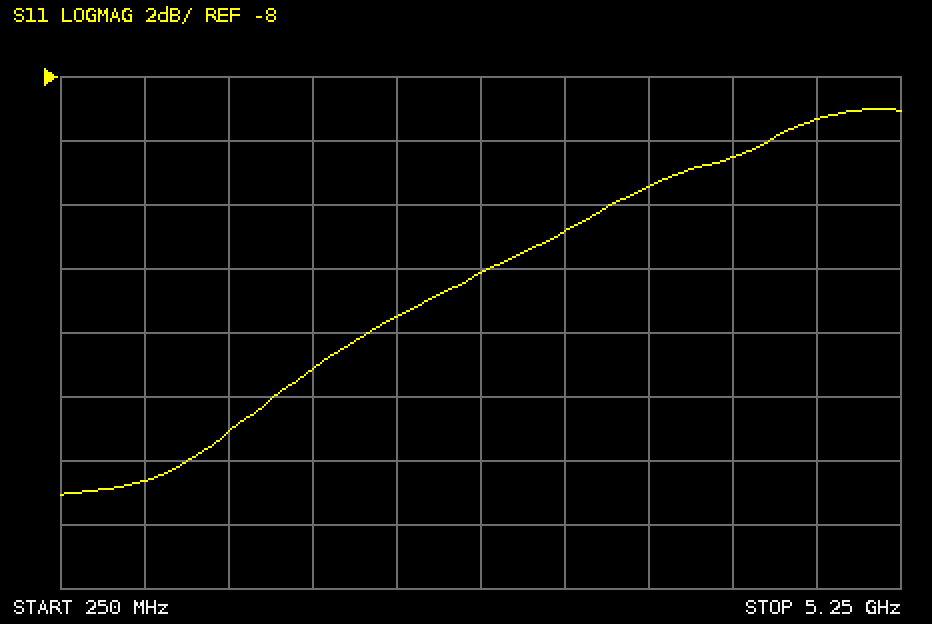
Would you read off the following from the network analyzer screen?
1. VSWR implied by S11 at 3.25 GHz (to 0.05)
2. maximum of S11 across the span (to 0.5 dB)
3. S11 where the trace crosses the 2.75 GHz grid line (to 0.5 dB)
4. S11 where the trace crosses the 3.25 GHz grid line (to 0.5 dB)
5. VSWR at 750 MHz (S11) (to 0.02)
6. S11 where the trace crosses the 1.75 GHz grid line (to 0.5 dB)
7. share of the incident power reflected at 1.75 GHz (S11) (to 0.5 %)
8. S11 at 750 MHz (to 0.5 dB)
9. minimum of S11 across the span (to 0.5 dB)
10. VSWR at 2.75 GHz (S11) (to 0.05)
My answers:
1.60
-9.0 dB
-14.0 dB
-13.0 dB
1.20
-17.0 dB
2.0 %
-20.5 dB
-21.0 dB
1.50
